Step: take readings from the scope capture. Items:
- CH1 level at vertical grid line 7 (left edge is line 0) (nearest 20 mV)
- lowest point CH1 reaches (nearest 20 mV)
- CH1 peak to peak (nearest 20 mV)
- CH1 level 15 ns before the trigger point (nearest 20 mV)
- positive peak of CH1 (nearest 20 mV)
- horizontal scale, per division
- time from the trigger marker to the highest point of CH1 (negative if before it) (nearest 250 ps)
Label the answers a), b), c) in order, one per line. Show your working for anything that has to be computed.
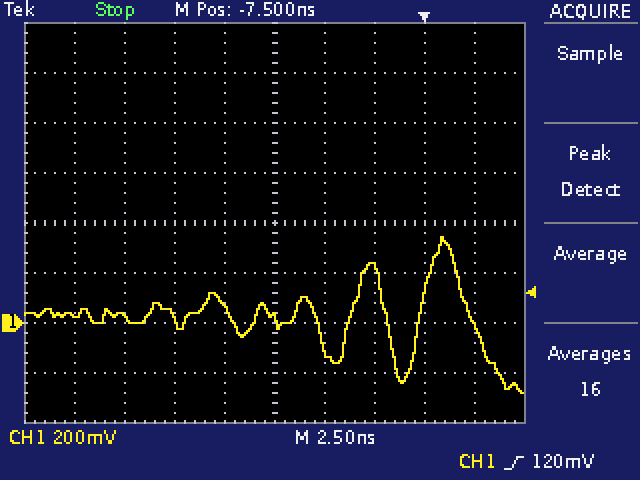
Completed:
a) 220 mV
b) -280 mV
c) 340 mV − (-280 mV) = 620 mV
d) 20 mV
e) 340 mV
f) 2.5 ns
g) +1.00 ns
